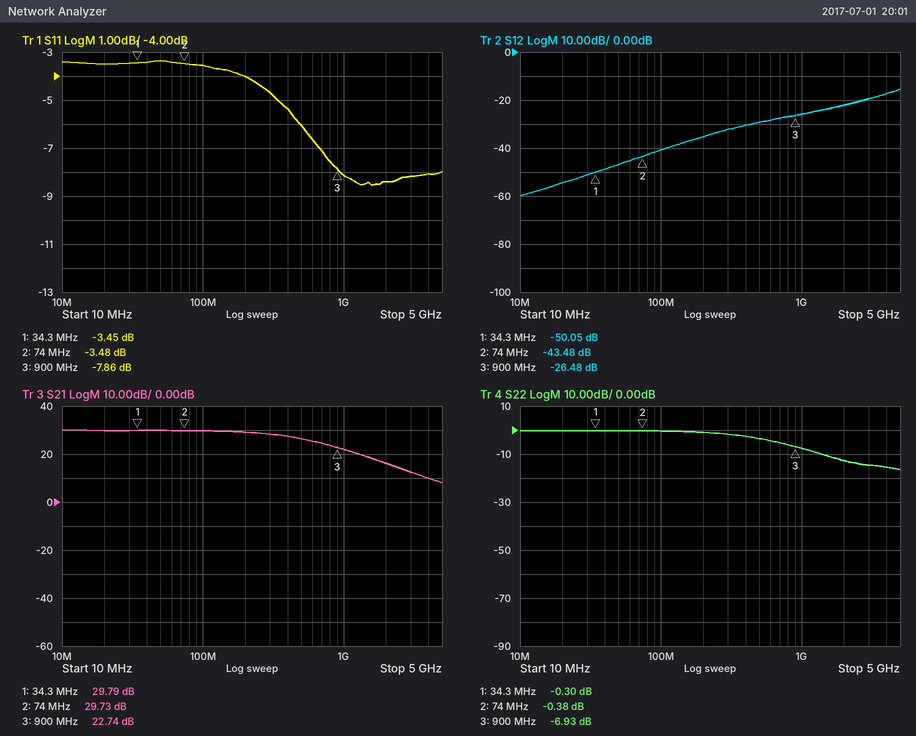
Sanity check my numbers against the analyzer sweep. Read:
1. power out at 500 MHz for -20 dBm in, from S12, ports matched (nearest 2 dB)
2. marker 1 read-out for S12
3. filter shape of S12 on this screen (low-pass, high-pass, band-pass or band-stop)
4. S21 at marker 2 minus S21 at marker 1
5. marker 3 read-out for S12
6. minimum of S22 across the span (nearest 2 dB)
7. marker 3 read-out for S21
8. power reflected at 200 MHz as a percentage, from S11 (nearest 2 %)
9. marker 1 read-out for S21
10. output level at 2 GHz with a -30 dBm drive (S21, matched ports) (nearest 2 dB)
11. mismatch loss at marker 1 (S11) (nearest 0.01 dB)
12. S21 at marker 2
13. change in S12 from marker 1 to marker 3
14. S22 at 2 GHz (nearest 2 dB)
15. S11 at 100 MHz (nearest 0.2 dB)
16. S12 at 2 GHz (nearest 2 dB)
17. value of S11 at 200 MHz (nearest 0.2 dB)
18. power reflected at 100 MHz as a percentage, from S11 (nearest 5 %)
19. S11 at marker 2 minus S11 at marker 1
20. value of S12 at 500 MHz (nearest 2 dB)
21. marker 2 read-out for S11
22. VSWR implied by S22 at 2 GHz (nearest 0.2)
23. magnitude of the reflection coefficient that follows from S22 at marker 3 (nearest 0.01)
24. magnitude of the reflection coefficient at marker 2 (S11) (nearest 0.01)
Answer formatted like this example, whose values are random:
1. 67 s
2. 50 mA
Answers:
1. -50 dBm
2. -50.05 dB
3. high-pass
4. -0.06 dB
5. -26.48 dB
6. -16 dB
7. 22.74 dB
8. 40 %
9. 29.79 dB
10. -14 dBm
11. 2.61 dB
12. 29.73 dB
13. 23.57 dB
14. -12 dB
15. -3.6 dB
16. -22 dB
17. -4.0 dB
18. 45 %
19. -0.03 dB
20. -30 dB
21. -3.48 dB
22. 1.6
23. 0.45
24. 0.67
